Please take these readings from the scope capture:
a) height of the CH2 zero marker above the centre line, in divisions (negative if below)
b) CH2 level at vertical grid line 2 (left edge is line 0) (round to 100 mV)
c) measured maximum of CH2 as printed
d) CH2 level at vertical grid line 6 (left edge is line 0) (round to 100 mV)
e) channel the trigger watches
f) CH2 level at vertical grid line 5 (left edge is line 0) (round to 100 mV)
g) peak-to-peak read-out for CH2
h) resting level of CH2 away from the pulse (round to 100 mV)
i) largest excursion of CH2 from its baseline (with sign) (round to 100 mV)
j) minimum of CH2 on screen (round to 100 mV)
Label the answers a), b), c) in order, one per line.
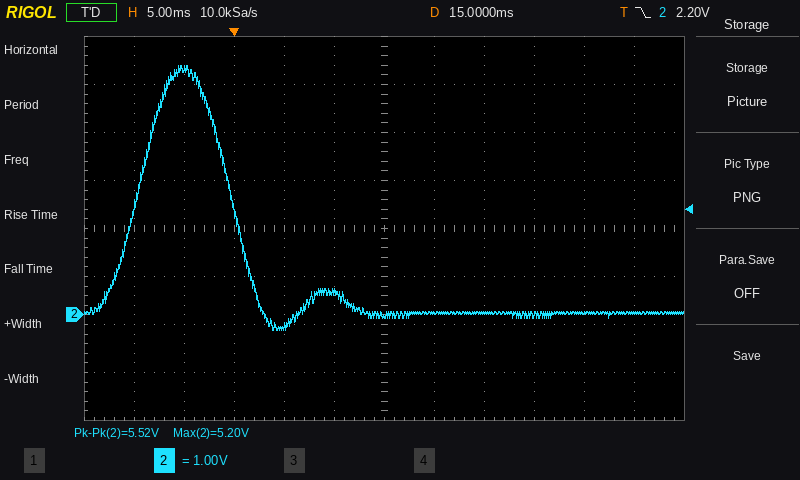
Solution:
a) -1.8 div
b) 5.1 V
c) 5.20 V
d) 0.0 V
e) CH2
f) 500 mV
g) 5.52 V
h) 0.0 V
i) +5.2 V
j) -300 mV
